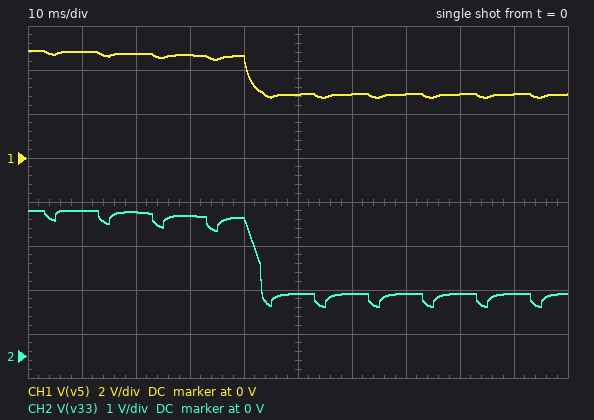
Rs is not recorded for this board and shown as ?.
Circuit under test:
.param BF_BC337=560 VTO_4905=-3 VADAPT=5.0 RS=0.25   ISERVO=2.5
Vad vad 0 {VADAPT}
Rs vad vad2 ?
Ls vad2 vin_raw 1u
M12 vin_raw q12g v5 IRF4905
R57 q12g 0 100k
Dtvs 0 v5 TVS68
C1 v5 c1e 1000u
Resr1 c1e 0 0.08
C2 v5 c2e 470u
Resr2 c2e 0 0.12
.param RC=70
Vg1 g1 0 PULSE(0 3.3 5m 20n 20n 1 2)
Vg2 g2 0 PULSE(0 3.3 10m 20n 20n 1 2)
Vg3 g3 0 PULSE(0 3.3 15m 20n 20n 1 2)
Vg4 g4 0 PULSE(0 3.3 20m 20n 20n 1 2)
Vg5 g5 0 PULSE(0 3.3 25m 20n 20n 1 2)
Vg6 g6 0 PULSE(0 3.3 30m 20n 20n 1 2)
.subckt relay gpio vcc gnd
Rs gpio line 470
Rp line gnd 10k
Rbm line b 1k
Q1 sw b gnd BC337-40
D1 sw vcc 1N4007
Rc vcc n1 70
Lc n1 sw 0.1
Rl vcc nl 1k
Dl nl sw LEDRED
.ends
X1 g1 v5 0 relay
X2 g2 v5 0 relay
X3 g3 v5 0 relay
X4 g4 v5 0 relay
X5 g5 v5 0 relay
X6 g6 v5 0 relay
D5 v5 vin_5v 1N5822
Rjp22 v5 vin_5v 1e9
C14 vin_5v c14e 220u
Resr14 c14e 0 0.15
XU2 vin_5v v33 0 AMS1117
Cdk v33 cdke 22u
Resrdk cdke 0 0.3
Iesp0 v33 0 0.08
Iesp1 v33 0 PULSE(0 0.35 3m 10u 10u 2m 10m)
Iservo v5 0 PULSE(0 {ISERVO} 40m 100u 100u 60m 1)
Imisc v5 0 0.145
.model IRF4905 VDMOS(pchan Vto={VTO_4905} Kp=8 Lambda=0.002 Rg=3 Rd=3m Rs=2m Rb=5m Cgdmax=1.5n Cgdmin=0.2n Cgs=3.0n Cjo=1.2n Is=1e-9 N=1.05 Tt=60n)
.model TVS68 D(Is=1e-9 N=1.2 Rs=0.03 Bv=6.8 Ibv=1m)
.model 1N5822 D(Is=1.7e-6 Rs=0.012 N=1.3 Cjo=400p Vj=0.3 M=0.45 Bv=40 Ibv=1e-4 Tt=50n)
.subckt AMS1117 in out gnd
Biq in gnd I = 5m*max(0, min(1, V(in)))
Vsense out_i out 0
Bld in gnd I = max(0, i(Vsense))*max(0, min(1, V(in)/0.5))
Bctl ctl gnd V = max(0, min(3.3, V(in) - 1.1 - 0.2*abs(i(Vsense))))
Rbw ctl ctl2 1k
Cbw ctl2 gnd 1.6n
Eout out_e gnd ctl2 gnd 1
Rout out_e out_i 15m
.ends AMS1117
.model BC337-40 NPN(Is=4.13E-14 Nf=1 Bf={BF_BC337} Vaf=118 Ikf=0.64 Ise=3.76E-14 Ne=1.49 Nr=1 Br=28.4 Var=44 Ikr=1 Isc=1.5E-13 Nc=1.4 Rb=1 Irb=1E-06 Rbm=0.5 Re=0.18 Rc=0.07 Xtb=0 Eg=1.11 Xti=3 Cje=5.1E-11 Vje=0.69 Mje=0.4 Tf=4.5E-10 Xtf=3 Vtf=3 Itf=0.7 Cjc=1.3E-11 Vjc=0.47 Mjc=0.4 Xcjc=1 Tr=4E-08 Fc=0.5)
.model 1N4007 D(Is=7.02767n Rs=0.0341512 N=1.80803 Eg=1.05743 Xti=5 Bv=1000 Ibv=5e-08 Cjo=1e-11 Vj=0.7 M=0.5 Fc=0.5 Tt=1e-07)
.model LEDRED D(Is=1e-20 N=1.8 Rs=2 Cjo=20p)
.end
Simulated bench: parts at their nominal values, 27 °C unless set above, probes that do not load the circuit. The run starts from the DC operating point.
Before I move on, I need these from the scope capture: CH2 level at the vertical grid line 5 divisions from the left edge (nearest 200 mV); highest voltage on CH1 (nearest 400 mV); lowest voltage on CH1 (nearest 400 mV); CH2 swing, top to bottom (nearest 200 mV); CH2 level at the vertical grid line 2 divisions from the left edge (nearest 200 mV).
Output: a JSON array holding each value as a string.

["1.4 V", "4.8 V", "2.8 V", "2.2 V", "3.2 V"]
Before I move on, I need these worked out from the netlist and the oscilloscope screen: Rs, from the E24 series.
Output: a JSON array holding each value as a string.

["0.51 Ω"]
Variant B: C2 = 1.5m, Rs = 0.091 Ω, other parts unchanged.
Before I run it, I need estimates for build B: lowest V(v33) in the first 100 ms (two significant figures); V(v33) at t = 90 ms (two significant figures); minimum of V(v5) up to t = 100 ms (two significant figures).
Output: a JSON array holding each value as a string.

["2.8 V", "3.0 V", "4.4 V"]
